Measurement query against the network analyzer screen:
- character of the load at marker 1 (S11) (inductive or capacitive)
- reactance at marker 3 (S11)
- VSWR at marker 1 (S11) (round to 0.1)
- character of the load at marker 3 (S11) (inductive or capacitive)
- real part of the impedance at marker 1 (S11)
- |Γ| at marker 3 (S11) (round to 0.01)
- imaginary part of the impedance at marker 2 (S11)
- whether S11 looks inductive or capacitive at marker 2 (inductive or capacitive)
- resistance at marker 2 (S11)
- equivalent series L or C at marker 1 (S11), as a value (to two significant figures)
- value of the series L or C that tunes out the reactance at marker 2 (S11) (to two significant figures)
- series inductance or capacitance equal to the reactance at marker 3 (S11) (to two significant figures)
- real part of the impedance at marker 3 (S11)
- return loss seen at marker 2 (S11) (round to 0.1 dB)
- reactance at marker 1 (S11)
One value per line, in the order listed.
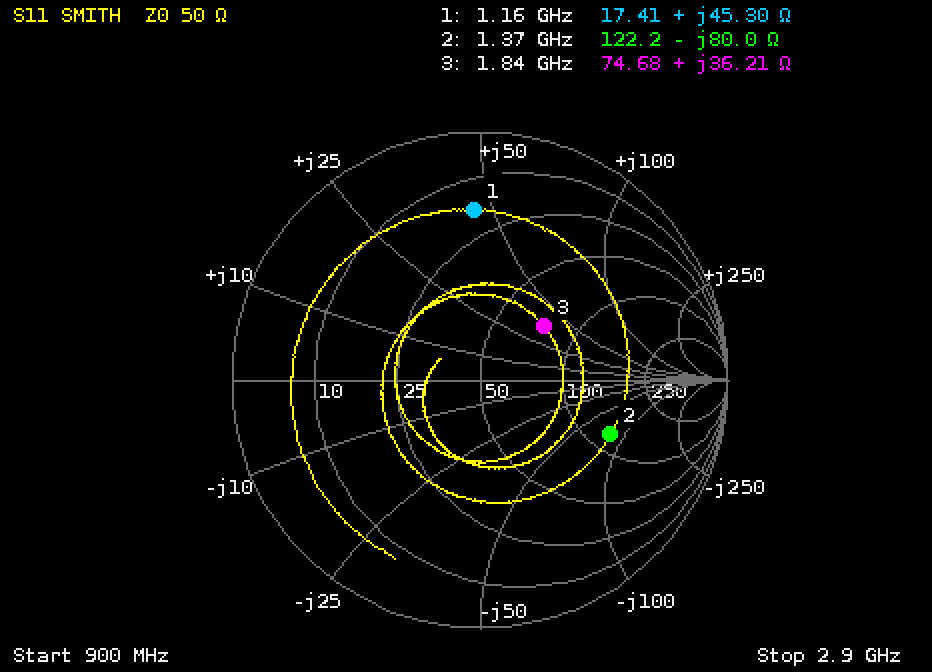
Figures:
inductive
+36.21 Ω
5.4
inductive
17.41 Ω
0.34
-80.0 Ω
capacitive
122.2 Ω
6.2 nH
9.3 nH
3.1 nH
74.68 Ω
4.9 dB
+45.30 Ω
